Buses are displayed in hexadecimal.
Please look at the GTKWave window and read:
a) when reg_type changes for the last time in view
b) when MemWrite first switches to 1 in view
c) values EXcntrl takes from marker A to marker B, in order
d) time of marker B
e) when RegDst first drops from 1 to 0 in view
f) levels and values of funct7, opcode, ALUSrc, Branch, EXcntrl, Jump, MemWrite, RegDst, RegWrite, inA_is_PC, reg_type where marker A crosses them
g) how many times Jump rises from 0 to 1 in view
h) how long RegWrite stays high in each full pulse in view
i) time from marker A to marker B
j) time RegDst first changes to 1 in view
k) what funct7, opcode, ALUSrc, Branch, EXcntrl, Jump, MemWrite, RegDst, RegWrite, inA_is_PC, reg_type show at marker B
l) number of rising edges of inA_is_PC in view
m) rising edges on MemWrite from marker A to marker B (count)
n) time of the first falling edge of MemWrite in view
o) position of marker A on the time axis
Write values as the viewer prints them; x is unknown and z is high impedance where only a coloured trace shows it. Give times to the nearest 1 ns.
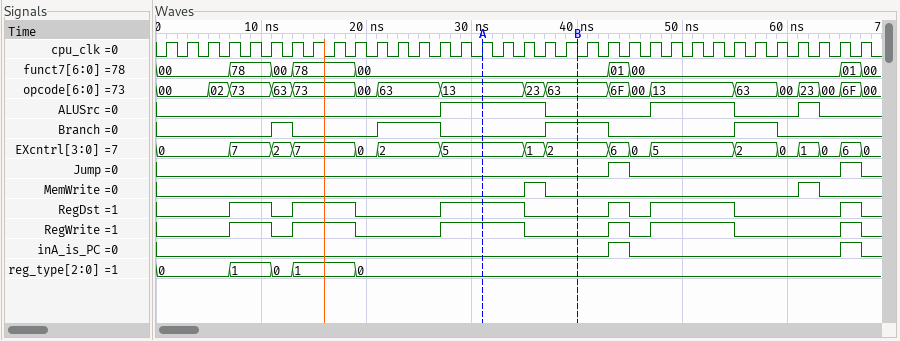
19 ns
35 ns
5, 1, 2
40 ns
11 ns
funct7=00, opcode=13, ALUSrc=1, Branch=0, EXcntrl=5, Jump=0, MemWrite=0, RegDst=1, RegWrite=1, inA_is_PC=0, reg_type=0
2
4 ns, 6 ns, 8 ns, 2 ns, 8 ns, 2 ns
9 ns
7 ns
funct7=00, opcode=63, ALUSrc=0, Branch=1, EXcntrl=2, Jump=0, MemWrite=0, RegDst=0, RegWrite=0, inA_is_PC=0, reg_type=0
2
1
37 ns
31 ns
